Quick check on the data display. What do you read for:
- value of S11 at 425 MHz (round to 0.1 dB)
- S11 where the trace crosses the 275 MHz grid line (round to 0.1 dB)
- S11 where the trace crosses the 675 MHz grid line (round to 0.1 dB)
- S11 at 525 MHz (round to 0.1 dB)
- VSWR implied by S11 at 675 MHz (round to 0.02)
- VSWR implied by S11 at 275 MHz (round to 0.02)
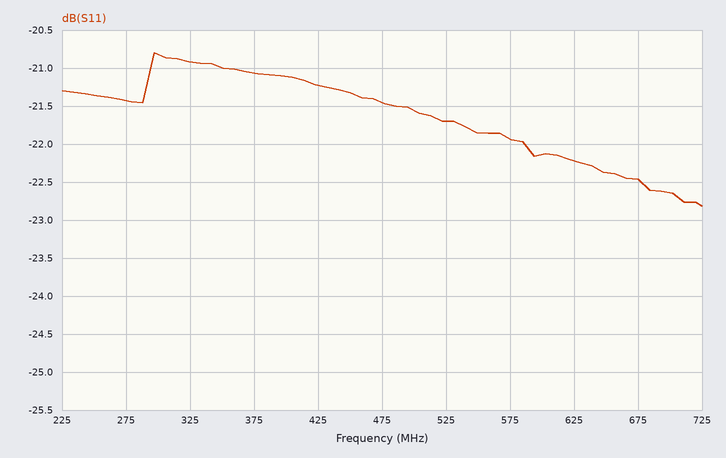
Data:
-21.2 dB
-21.4 dB
-22.5 dB
-21.7 dB
1.16
1.18
